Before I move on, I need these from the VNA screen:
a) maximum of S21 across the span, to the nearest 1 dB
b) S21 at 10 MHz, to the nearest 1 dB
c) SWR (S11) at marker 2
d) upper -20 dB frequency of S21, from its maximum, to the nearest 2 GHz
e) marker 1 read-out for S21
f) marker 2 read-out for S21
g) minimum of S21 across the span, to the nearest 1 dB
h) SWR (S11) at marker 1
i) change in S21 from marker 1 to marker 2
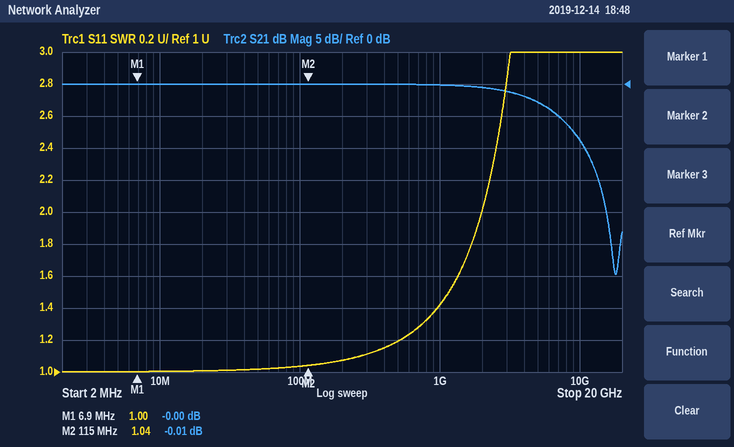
0 dB
0 dB
1.04
16 GHz
-0.00 dB
-0.01 dB
-30 dB
1.00
-0.01 dB
